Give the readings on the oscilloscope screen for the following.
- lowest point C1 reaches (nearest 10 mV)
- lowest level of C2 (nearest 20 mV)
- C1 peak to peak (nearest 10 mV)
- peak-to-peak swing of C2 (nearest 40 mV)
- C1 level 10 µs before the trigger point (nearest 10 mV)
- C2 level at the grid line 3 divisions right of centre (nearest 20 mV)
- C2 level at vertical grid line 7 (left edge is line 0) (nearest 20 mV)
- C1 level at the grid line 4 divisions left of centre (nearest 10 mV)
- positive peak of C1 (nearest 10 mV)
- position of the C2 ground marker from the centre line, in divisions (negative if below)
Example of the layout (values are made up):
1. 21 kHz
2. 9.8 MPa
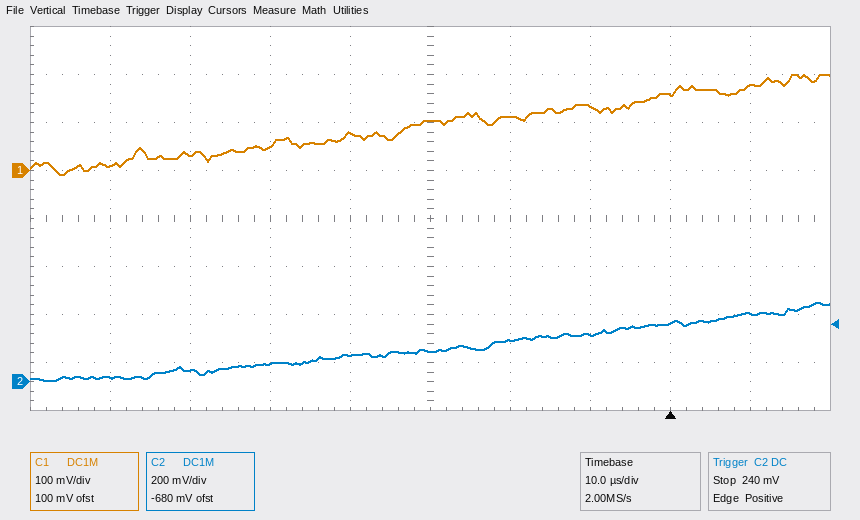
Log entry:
1. -10 mV
2. 0 mV
3. 210 mV
4. 320 mV
5. 130 mV
6. 240 mV
7. 200 mV
8. 10 mV
9. 200 mV
10. -3.4 div
